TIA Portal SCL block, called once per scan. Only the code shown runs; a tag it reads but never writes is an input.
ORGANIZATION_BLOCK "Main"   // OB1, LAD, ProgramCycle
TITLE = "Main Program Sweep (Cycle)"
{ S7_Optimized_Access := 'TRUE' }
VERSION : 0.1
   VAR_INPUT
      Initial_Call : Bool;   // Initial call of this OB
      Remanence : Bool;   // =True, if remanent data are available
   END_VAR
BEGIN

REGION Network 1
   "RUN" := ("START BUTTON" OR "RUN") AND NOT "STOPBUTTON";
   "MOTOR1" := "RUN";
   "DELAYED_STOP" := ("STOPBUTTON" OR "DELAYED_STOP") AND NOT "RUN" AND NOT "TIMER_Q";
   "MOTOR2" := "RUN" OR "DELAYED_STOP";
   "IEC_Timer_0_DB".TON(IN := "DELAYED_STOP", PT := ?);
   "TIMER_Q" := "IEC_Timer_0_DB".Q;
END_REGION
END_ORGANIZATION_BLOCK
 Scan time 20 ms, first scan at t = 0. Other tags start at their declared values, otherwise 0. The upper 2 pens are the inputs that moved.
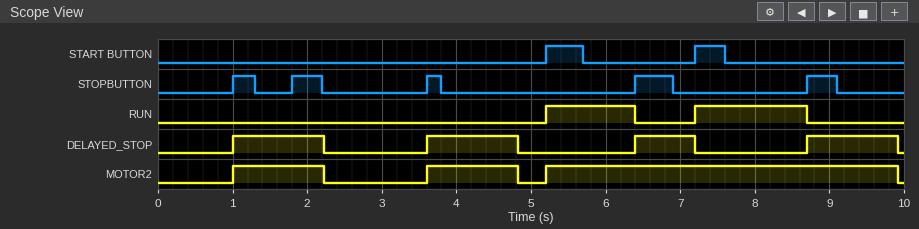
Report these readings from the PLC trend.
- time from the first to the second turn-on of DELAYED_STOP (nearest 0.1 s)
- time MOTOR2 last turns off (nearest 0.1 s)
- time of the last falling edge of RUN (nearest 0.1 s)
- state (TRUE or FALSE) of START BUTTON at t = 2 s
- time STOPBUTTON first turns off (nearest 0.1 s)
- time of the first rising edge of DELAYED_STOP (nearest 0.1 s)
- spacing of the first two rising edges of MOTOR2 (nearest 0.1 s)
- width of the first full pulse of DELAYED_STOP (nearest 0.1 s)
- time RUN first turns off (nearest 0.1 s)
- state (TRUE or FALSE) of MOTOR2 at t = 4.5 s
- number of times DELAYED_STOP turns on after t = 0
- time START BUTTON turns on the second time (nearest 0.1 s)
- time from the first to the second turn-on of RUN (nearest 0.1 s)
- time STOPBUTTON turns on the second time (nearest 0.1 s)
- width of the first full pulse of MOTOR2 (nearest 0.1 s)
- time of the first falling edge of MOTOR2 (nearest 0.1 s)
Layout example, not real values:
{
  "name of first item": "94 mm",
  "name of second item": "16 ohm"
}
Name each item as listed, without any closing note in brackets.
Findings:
{
  "time from the first to the second turn-on of DELAYED_STOP": "2.6 s",
  "time MOTOR2 last turns off": "9.9 s",
  "time of the last falling edge of RUN": "8.7 s",
  "state (TRUE or FALSE) of START BUTTON at t = 2 s": "FALSE",
  "time STOPBUTTON first turns off": "1.3 s",
  "time of the first rising edge of DELAYED_STOP": "1.0 s",
  "spacing of the first two rising edges of MOTOR2": "2.6 s",
  "width of the first full pulse of DELAYED_STOP": "1.2 s",
  "time RUN first turns off": "6.4 s",
  "state (TRUE or FALSE) of MOTOR2 at t = 4.5 s": "TRUE",
  "number of times DELAYED_STOP turns on after t = 0": "4",
  "time START BUTTON turns on the second time": "7.2 s",
  "time from the first to the second turn-on of RUN": "2.0 s",
  "time STOPBUTTON turns on the second time": "1.8 s",
  "width of the first full pulse of MOTOR2": "1.2 s",
  "time of the first falling edge of MOTOR2": "2.2 s"
}
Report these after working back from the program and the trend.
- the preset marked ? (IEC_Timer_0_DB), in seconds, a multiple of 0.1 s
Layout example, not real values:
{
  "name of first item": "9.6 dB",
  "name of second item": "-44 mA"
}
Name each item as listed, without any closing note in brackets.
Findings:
{
  "the preset marked ? (IEC_Timer_0_DB), in seconds, a multiple of 0.1 s": "1.2 s"
}
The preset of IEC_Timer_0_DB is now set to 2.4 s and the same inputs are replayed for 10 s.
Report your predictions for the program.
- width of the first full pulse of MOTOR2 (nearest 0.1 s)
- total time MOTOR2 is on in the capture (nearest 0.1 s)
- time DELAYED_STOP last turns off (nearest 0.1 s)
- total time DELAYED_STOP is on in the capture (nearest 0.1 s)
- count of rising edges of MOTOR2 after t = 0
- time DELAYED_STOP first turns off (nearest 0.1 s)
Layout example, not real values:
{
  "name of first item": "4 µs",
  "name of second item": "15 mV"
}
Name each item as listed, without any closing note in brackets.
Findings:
{
  "width of the first full pulse of MOTOR2": "2.4 s",
  "total time MOTOR2 is on in the capture": "8.8 s",
  "time DELAYED_STOP last turns off": "7.2 s",
  "total time DELAYED_STOP is on in the capture": "6.1 s",
  "count of rising edges of MOTOR2 after t = 0": "2",
  "time DELAYED_STOP first turns off": "3.4 s"
}
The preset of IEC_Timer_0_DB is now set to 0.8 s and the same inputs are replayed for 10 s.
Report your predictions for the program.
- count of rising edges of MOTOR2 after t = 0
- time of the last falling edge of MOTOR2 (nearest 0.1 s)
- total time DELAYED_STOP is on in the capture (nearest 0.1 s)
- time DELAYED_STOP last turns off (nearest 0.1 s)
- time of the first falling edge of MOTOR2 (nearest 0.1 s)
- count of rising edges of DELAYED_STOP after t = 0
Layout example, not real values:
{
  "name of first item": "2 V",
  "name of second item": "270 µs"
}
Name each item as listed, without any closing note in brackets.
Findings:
{
  "count of rising edges of MOTOR2 after t = 0": "4",
  "time of the last falling edge of MOTOR2": "9.5 s",
  "total time DELAYED_STOP is on in the capture": "4.1 s",
  "time DELAYED_STOP last turns off": "9.5 s",
  "time of the first falling edge of MOTOR2": "1.8 s",
  "count of rising edges of DELAYED_STOP after t = 0": "5"
}
